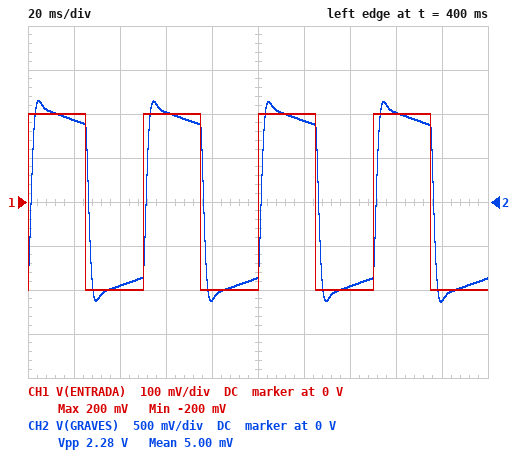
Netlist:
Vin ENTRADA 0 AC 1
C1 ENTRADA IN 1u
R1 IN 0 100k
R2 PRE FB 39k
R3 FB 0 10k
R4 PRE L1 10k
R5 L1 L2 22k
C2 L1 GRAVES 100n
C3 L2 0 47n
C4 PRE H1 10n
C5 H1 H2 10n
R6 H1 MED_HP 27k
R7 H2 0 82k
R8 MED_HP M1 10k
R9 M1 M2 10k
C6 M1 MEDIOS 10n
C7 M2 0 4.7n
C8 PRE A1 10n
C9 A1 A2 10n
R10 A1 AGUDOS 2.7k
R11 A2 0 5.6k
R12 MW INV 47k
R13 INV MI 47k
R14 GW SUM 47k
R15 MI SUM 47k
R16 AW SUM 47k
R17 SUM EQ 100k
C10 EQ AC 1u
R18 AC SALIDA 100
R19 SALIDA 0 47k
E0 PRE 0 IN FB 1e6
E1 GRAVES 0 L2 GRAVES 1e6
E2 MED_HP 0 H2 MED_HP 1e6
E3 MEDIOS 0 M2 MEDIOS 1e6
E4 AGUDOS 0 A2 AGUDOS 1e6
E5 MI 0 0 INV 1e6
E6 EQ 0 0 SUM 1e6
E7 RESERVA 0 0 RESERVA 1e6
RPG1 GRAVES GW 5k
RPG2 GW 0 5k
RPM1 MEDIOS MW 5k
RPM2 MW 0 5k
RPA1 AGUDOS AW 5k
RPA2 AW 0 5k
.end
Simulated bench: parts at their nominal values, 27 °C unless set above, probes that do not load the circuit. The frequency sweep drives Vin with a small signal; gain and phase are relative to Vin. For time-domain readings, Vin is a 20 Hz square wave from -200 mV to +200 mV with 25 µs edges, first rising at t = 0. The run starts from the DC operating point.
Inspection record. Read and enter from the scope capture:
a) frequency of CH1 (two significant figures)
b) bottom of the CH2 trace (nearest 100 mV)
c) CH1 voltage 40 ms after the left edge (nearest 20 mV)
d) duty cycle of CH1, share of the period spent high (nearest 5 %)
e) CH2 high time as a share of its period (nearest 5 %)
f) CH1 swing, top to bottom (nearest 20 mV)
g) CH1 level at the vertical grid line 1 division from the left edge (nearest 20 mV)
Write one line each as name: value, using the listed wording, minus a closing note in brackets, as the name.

frequency of CH1: 20 Hz
bottom of the CH2 trace: -1.1 V
CH1 voltage 40 ms after the left edge: -200 mV
duty cycle of CH1, share of the period spent high: 50 %
CH2 high time as a share of its period: 50 %
CH1 swing, top to bottom: 400 mV
CH1 level at the vertical grid line 1 division from the left edge: 200 mV
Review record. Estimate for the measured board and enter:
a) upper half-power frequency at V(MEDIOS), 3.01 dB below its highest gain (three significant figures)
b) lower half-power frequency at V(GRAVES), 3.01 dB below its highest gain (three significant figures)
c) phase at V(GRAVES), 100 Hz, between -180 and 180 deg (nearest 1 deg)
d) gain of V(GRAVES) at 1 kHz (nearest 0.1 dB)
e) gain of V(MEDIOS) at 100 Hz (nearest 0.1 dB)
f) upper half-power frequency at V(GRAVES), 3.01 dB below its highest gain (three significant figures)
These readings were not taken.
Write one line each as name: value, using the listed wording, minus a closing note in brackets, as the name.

upper half-power frequency at V(MEDIOS), 3.01 dB below its highest gain: 2.26 kHz
lower half-power frequency at V(GRAVES), 3.01 dB below its highest gain: 1.58 Hz
phase at V(GRAVES), 100 Hz, between -180 and 180 deg: -57 deg
gain of V(GRAVES) at 1 kHz: -18.4 dB
gain of V(MEDIOS) at 100 Hz: -7.1 dB
upper half-power frequency at V(GRAVES), 3.01 dB below its highest gain: 150 Hz
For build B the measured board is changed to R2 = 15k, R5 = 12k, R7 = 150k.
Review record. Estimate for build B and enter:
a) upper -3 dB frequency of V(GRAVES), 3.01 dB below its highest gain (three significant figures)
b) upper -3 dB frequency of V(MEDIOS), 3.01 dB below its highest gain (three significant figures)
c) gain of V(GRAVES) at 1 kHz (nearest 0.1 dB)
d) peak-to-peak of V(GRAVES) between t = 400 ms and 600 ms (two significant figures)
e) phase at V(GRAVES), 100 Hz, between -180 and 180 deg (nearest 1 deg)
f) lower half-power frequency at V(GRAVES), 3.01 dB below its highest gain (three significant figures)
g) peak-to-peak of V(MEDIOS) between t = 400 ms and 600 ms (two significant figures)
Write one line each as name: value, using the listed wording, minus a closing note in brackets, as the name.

upper -3 dB frequency of V(GRAVES), 3.01 dB below its highest gain: 217 Hz
upper -3 dB frequency of V(MEDIOS), 3.01 dB below its highest gain: 1.68 kHz
gain of V(GRAVES) at 1 kHz: -19.0 dB
peak-to-peak of V(GRAVES) between t = 400 ms and 600 ms: 1.2 V
phase at V(GRAVES), 100 Hz, between -180 and 180 deg: -39 deg
lower half-power frequency at V(GRAVES), 3.01 dB below its highest gain: 1.59 Hz
peak-to-peak of V(MEDIOS) between t = 400 ms and 600 ms: 1.7 V
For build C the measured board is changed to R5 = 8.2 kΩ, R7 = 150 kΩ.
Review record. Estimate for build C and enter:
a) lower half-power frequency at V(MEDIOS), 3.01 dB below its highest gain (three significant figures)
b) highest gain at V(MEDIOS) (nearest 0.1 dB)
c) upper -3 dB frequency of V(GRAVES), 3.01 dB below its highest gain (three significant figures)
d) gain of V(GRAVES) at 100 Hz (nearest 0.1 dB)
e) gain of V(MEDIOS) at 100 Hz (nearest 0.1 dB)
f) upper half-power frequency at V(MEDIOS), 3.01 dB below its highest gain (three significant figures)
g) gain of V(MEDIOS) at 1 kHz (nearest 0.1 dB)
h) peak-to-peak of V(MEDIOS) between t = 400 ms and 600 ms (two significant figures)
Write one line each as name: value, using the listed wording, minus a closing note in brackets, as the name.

lower half-power frequency at V(MEDIOS), 3.01 dB below its highest gain: 211 Hz
highest gain at V(MEDIOS): 16.1 dB
upper -3 dB frequency of V(GRAVES), 3.01 dB below its highest gain: 263 Hz
gain of V(GRAVES) at 100 Hz: 13.8 dB
gain of V(MEDIOS) at 100 Hz: -1.3 dB
upper half-power frequency at V(MEDIOS), 3.01 dB below its highest gain: 1.68 kHz
gain of V(MEDIOS) at 1 kHz: 14.1 dB
peak-to-peak of V(MEDIOS) between t = 400 ms and 600 ms: 3.3 V
